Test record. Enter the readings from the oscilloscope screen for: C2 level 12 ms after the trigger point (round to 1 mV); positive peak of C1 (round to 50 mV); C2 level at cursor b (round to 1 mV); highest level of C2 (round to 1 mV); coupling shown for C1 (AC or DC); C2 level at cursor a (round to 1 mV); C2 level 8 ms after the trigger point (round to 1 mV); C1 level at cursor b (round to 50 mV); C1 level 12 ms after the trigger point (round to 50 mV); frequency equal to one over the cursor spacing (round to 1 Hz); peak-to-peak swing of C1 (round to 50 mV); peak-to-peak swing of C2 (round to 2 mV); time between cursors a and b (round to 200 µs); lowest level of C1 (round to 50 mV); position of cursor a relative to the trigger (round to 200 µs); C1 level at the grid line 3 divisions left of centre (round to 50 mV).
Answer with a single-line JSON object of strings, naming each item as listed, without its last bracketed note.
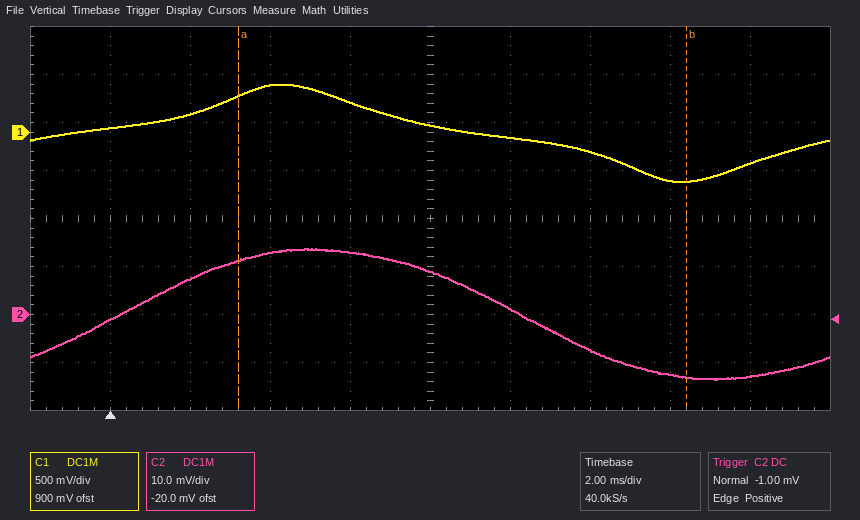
{"C2 level 12 ms after the trigger point": "-7 mV", "positive peak of C1": "500 mV", "C2 level at cursor b": "-13 mV", "highest level of C2": "14 mV", "coupling shown for C1": "DC", "C2 level at cursor a": "11 mV", "C2 level 8 ms after the trigger point": "9 mV", "C1 level at cursor b": "-500 mV", "C1 level 12 ms after the trigger point": "-200 mV", "frequency equal to one over the cursor spacing": "89 Hz", "peak-to-peak swing of C1": "1.00 V", "peak-to-peak swing of C2": "28 mV", "time between cursors a and b": "11.2 ms", "lowest level of C1": "-500 mV", "position of cursor a relative to the trigger": "+3.2 ms", "C1 level at the grid line 3 divisions left of centre": "200 mV"}
